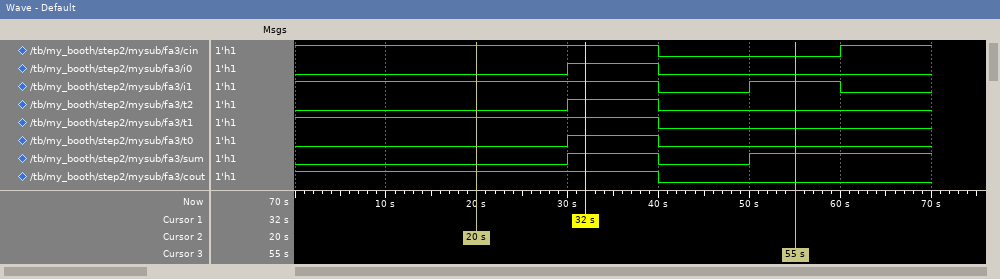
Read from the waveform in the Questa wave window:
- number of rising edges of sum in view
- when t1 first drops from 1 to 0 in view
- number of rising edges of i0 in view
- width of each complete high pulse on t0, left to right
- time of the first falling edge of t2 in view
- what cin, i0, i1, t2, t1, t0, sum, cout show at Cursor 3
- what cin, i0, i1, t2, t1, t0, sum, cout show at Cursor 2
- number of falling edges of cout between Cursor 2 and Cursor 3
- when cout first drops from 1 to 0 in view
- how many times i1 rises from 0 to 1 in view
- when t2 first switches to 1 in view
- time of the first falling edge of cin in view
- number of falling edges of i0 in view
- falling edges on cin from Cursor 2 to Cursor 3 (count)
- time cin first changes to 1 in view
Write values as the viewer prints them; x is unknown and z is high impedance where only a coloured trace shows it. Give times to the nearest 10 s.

2
40 s
1
10 s
40 s
cin=0, i0=0, i1=1, t2=0, t1=0, t0=0, sum=1, cout=0
cin=1, i0=0, i1=1, t2=0, t1=1, t0=0, sum=0, cout=1
1
40 s
1
30 s
40 s
1
1
60 s
